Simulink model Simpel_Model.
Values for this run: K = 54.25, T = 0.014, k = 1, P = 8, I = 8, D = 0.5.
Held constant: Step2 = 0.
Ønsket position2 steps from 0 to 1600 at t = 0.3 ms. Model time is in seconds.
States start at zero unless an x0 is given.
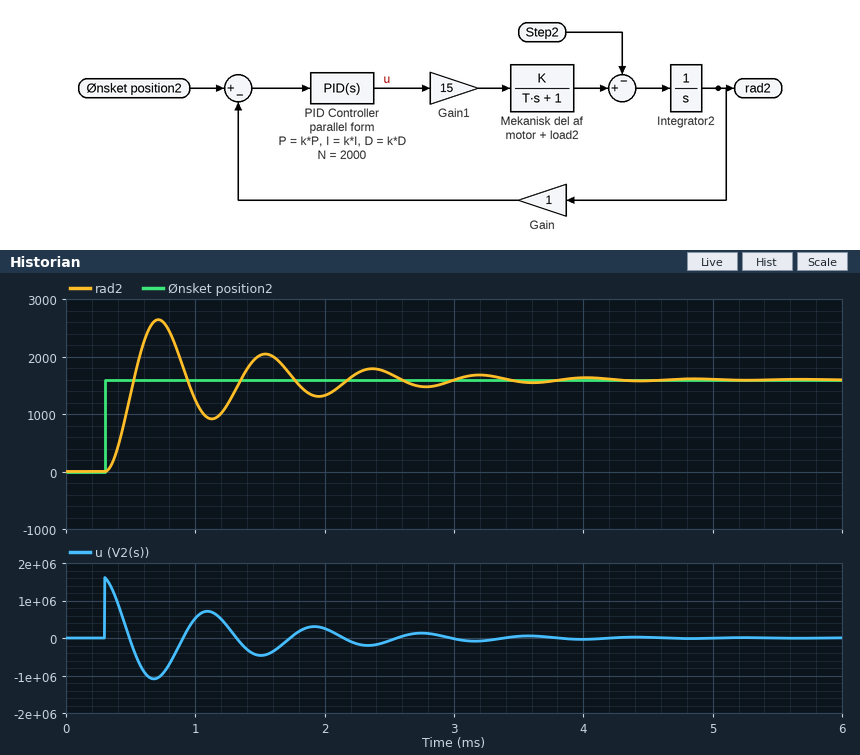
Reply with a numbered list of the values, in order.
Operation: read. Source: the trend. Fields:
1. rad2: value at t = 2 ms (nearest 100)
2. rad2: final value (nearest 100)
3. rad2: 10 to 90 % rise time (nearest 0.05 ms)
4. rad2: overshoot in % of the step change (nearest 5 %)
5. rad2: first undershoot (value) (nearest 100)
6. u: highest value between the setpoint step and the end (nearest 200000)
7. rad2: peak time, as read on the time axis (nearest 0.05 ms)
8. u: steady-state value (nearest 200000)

1. 1300
2. 1600
3. 0.15 ms
4. 65 %
5. 900
6. 1600000
7. 0.70 ms
8. 0
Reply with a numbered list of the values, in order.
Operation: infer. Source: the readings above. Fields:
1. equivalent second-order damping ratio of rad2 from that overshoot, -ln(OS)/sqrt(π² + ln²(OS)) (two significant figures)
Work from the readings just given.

1. 0.14
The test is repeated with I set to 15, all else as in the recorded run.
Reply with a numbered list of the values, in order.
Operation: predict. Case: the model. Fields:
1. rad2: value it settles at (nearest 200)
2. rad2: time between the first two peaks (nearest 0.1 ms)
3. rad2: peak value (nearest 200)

1. 1600
2. 0.8 ms
3. 2600
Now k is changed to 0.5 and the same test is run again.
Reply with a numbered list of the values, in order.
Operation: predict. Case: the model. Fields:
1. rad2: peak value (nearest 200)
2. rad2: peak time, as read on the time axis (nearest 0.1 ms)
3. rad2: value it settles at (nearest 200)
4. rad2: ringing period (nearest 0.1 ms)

1. 2400
2. 0.9 ms
3. 1600
4. 1.2 ms
